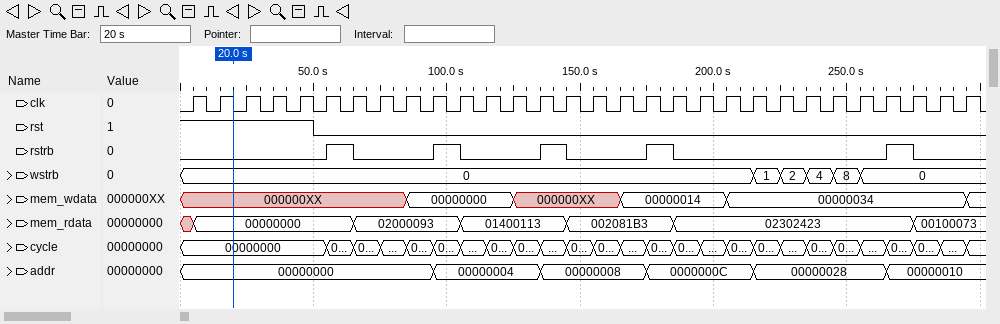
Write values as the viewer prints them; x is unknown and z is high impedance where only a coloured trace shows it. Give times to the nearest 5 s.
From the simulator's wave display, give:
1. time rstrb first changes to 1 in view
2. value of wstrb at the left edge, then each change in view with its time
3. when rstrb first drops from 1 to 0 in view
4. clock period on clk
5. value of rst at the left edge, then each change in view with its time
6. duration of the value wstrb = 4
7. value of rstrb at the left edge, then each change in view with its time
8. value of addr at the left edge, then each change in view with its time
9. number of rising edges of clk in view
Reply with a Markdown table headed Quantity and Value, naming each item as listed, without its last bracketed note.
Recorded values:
| Quantity | Value |
|---|---|
| time rstrb first changes to 1 in view | 55 s |
| value of wstrb at the left edge, then each change in view with its time | 0, 1 at 215 s, 2 at 225 s, 4 at 235 s, 8 at 245 s, 0 at 255 s |
| when rstrb first drops from 1 to 0 in view | 65 s |
| clock period on clk | 10 s |
| value of rst at the left edge, then each change in view with its time | 1, 0 at 50 s |
| duration of the value wstrb = 4 | 10 s |
| value of rstrb at the left edge, then each change in view with its time | 0, 1 at 55 s, 0 at 65 s, 1 at 95 s, 0 at 105 s, 1 at 135 s, 0 at 145 s, 1 at 175 s, 0 at 185 s, 1 at 265 s, 0 at 275 s |
| value of addr at the left edge, then each change in view with its time | 00000000, 00000004 at 95 s, 00000008 at 135 s, 0000000C at 175 s, 00000028 at 215 s, 00000010 at 265 s |
| number of rising edges of clk in view | 30 |
